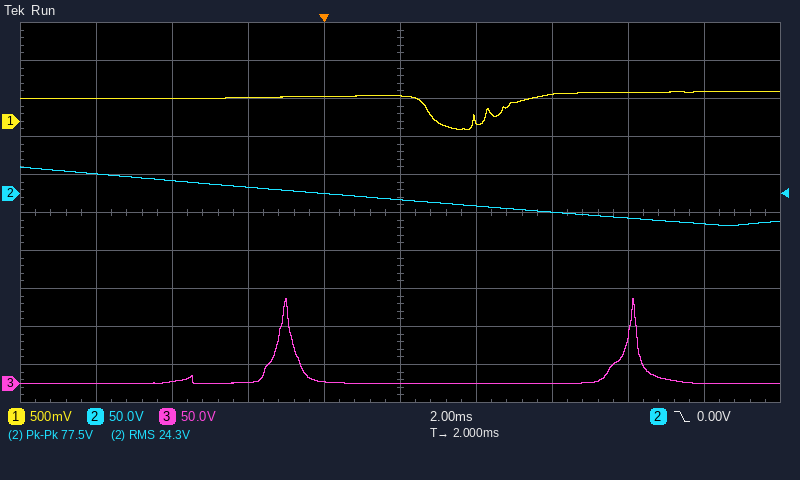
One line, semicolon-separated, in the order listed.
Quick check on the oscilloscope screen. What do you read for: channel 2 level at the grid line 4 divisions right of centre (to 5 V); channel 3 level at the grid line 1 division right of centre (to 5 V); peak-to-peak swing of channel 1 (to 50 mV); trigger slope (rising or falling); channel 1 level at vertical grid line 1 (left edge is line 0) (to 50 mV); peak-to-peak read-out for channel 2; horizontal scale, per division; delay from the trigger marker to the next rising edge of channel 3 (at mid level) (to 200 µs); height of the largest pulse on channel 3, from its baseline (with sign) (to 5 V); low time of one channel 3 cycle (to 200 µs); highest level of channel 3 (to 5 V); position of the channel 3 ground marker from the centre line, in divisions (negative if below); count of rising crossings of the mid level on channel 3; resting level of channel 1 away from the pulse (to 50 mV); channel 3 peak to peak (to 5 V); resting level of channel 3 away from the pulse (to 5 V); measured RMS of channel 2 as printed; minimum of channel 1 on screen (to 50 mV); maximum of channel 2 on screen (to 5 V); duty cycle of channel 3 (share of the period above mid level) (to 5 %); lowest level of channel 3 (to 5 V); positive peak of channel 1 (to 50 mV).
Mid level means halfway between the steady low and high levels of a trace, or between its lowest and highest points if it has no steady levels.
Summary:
-40 V; 0 V; 500 mV; falling; 300 mV; 77.5 V; 2 ms; 8.0 ms; +110 V; 8.8 ms; 110 V; -4.5 div; 2; 300 mV; 110 V; 0 V; 24.3 V; -100 mV; 35 V; 5 %; 0 V; 400 mV
